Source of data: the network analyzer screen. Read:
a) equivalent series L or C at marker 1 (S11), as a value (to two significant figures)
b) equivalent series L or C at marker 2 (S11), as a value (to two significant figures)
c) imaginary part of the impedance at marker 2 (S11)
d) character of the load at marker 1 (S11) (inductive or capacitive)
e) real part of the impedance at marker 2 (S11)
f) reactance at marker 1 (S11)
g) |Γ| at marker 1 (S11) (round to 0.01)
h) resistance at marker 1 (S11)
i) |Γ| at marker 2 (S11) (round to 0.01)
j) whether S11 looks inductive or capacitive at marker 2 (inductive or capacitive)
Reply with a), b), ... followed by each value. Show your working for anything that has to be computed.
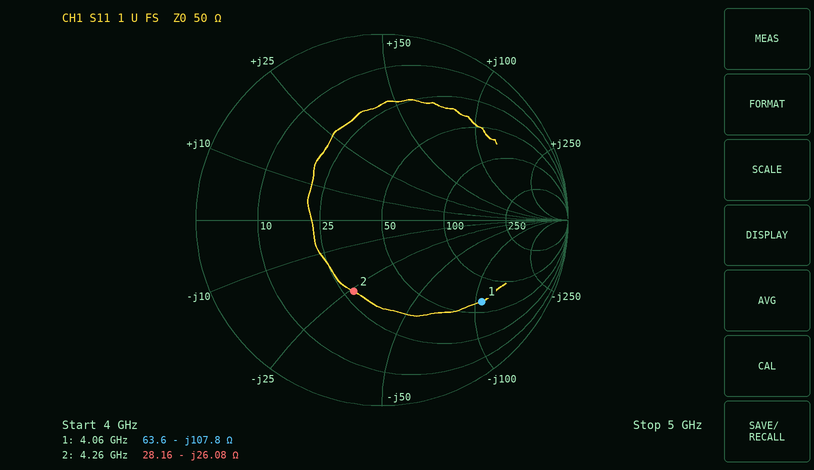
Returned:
a) C = 1/(2π × 4.06 GHz × 107.8 Ω) ≈ 364 fF, so 360 fF to two significant figures
b) C = 1/(2π × 4.26 GHz × 26.08 Ω) ≈ 1.4 pF
c) -26.08 Ω
d) capacitive
e) 28.16 Ω
f) -107.8 Ω
g) 0.69
h) 63.6 Ω
i) 0.41
j) capacitive
